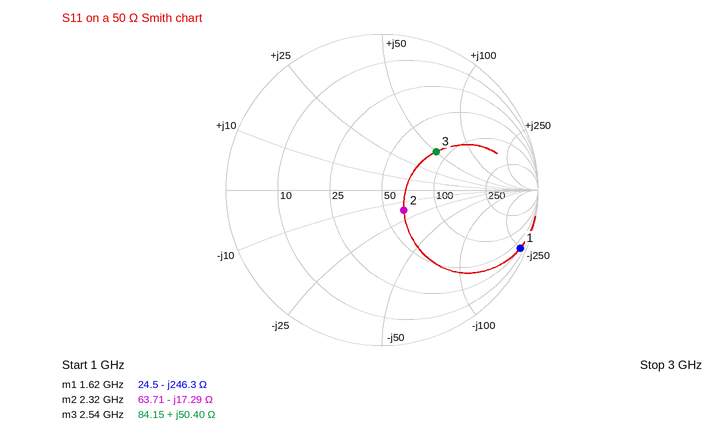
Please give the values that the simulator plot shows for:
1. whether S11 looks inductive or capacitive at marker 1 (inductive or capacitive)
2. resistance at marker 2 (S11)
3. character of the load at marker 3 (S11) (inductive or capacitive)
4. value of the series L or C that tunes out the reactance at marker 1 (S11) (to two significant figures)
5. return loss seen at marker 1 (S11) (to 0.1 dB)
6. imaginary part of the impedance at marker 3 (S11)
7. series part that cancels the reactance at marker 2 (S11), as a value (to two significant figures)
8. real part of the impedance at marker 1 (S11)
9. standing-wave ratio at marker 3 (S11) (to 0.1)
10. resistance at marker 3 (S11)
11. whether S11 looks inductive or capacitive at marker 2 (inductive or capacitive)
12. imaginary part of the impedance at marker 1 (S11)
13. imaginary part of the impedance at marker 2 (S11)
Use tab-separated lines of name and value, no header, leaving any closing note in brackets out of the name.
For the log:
whether S11 looks inductive or capacitive at marker 1	capacitive
resistance at marker 2	63.71 Ω
character of the load at marker 3 (S11)	inductive
value of the series L or C that tunes out the reactance at marker 1 (S11)	24 nH
return loss seen at marker 1 (S11)	0.3 dB
imaginary part of the impedance at marker 3	+50.40 Ω
series part that cancels the reactance at marker 2 (S11), as a value	1.2 nH
real part of the impedance at marker 1	24.5 Ω
standing-wave ratio at marker 3 (S11)	2.5
resistance at marker 3	84.15 Ω
whether S11 looks inductive or capacitive at marker 2	capacitive
imaginary part of the impedance at marker 1	-246.3 Ω
imaginary part of the impedance at marker 2	-17.29 Ω
